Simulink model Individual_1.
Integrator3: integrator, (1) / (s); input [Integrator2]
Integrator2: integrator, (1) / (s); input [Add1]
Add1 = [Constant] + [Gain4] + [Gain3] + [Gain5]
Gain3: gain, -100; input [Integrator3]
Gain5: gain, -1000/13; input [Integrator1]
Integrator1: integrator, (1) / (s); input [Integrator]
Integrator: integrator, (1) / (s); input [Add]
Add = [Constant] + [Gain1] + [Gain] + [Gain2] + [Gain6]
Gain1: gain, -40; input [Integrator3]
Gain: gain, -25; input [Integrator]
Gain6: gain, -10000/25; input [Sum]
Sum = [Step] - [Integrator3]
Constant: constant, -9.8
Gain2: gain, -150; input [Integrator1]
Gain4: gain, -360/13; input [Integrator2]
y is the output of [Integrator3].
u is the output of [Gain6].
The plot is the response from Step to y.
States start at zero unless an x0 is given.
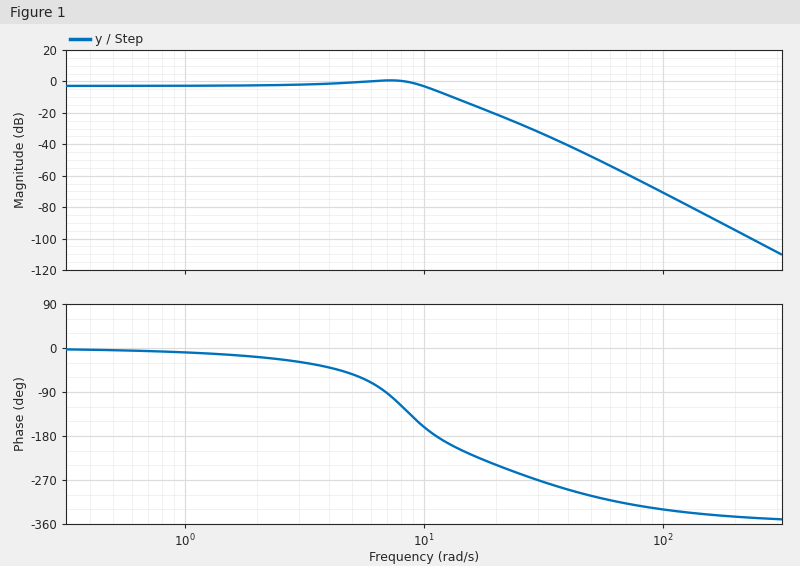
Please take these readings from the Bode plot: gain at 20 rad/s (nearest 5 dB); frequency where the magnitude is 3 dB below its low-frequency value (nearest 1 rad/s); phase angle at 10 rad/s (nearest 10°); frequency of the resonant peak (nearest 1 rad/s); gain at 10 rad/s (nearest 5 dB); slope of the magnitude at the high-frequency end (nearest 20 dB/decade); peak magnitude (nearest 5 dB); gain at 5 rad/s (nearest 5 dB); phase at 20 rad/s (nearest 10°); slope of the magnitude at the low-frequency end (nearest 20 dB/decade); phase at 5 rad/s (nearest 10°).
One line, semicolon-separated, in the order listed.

-20 dB; 11 rad/s; -160°; 7 rad/s; -5 dB; -80 dB/decade; 0 dB; 0 dB; -240°; 0 dB/decade; -50°
